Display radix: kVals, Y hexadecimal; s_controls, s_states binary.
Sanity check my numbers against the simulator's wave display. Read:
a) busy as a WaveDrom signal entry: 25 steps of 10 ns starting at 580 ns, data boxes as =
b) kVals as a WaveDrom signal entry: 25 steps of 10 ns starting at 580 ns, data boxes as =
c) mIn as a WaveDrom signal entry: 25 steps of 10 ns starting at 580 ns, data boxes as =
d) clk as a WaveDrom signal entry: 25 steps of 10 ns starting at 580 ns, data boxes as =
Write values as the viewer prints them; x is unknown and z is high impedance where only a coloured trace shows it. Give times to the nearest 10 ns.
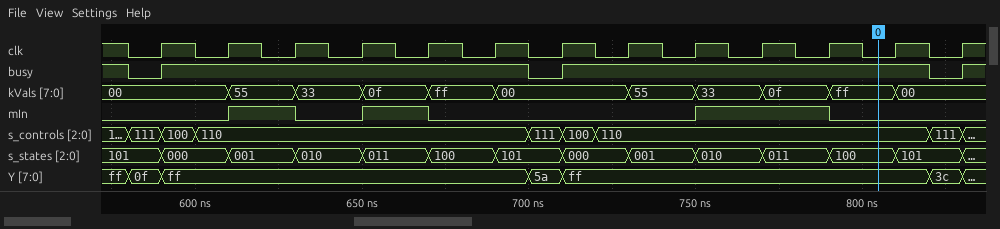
{name: 'busy', wave: '01..........01..........0'}
{name: 'kVals', wave: '=..=.=.=.=.=...=.=.=.=.=.', data: '00 55 33 0f ff 00 55 33 0f ff 00'}
{name: 'mIn', wave: '0..1.0.1.0.......1...0...'}
{name: 'clk', wave: '0101010101010101010101010'}
